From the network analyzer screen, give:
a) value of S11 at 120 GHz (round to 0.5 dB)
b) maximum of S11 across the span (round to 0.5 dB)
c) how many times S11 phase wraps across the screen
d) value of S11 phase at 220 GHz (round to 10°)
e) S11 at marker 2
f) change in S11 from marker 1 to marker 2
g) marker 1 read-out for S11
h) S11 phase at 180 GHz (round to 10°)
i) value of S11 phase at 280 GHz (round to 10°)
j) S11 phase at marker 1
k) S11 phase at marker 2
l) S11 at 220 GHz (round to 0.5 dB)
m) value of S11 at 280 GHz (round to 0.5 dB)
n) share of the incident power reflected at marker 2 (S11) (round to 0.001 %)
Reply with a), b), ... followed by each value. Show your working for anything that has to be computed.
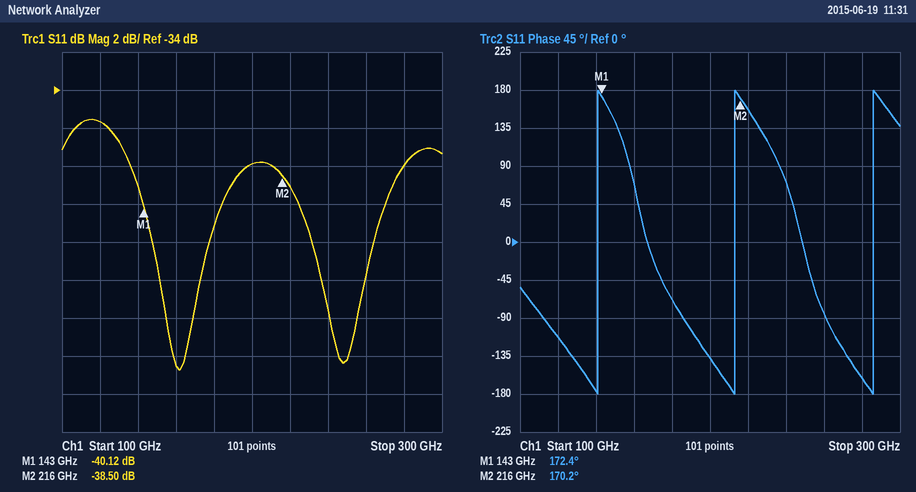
a) -35.5 dB
b) -35.5 dB
c) 3
d) 160°
e) -38.50 dB
f) -38.5 − (-40.12) = 1.62 dB
g) -40.12 dB
h) -70°
i) -160°
j) 172.4°
k) 170.2°
l) -39.0 dB
m) -38.0 dB
n) 10^(-38.5/10) ≈ 0.014 %
